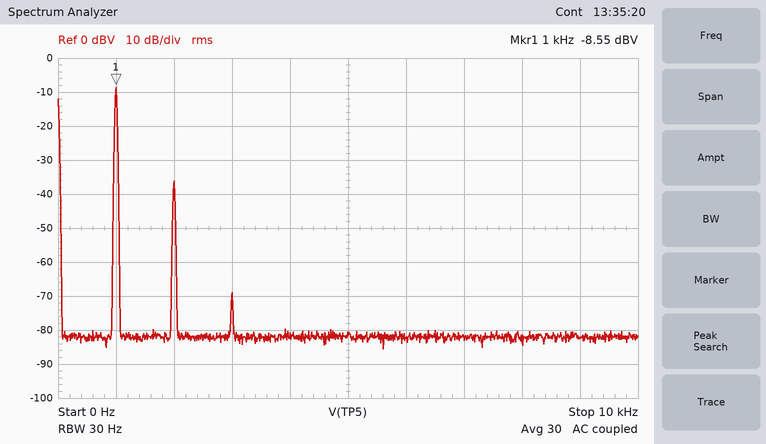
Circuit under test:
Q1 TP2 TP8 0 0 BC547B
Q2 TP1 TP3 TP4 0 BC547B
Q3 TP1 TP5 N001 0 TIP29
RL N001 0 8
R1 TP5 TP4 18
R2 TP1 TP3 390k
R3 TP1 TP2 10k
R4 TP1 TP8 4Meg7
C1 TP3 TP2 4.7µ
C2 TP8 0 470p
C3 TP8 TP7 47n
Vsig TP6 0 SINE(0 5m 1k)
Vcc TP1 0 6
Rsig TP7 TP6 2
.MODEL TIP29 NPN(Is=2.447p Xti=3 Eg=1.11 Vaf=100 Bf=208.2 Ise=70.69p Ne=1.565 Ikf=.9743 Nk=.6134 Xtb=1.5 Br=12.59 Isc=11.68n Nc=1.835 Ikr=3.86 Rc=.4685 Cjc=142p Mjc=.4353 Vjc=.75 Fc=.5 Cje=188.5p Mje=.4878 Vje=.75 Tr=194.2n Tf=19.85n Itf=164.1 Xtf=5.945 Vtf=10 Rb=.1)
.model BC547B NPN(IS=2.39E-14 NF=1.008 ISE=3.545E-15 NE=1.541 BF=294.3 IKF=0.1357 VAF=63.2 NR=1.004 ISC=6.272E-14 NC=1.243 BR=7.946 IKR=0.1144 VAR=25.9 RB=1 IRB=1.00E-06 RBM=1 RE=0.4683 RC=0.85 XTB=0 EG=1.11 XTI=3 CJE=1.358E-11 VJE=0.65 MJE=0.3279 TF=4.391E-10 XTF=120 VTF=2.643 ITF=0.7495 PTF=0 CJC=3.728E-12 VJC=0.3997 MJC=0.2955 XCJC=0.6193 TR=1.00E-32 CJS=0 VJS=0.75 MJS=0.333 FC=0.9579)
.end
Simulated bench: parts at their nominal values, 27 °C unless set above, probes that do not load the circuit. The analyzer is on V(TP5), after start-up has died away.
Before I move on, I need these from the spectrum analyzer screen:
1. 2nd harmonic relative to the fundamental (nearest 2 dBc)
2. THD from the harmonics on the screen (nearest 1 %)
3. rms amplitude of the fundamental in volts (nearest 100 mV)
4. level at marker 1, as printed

-28 dBc
4 %
400 mV
-8.55 dBV
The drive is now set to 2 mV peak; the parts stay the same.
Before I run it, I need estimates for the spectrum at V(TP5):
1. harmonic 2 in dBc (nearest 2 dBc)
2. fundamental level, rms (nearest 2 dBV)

-36 dBc
-16 dBV
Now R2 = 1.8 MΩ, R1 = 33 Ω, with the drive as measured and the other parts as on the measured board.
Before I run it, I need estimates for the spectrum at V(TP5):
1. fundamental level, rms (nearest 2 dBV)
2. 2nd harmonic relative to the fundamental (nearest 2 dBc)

-8 dBV
-30 dBc
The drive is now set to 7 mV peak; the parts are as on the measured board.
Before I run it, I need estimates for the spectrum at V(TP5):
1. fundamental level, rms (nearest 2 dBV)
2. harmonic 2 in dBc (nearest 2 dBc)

-6 dBV
-24 dBc
